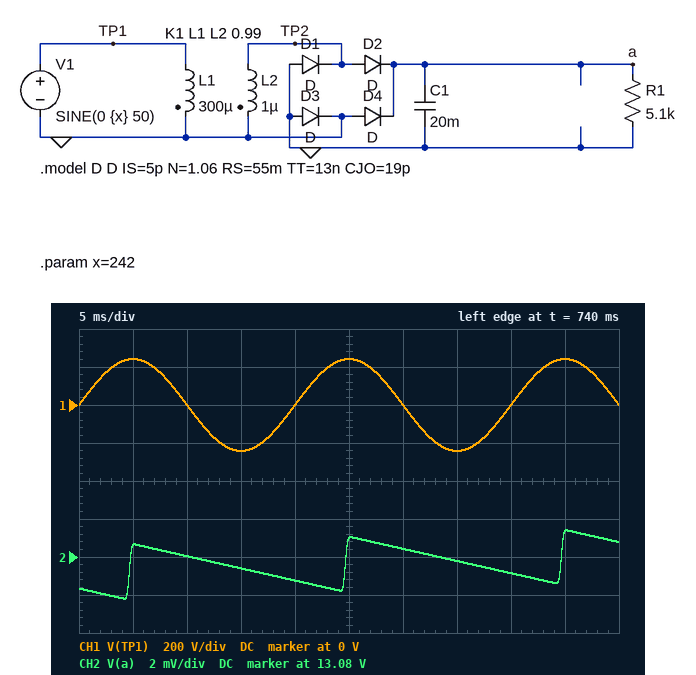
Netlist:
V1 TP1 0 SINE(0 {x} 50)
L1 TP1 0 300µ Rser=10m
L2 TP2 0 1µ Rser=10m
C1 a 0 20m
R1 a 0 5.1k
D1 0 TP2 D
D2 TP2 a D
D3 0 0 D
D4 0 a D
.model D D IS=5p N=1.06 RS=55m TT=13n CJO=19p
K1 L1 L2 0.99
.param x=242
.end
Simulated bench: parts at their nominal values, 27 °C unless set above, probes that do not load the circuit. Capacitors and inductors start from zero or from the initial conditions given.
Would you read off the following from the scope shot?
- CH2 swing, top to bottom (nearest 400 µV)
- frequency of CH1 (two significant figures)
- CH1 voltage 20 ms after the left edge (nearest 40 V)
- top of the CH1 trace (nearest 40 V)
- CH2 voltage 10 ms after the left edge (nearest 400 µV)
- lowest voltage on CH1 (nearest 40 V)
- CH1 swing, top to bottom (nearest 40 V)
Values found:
3.6 mV
50 Hz
0 V
240 V
13.0820 V
-240 V
480 V
